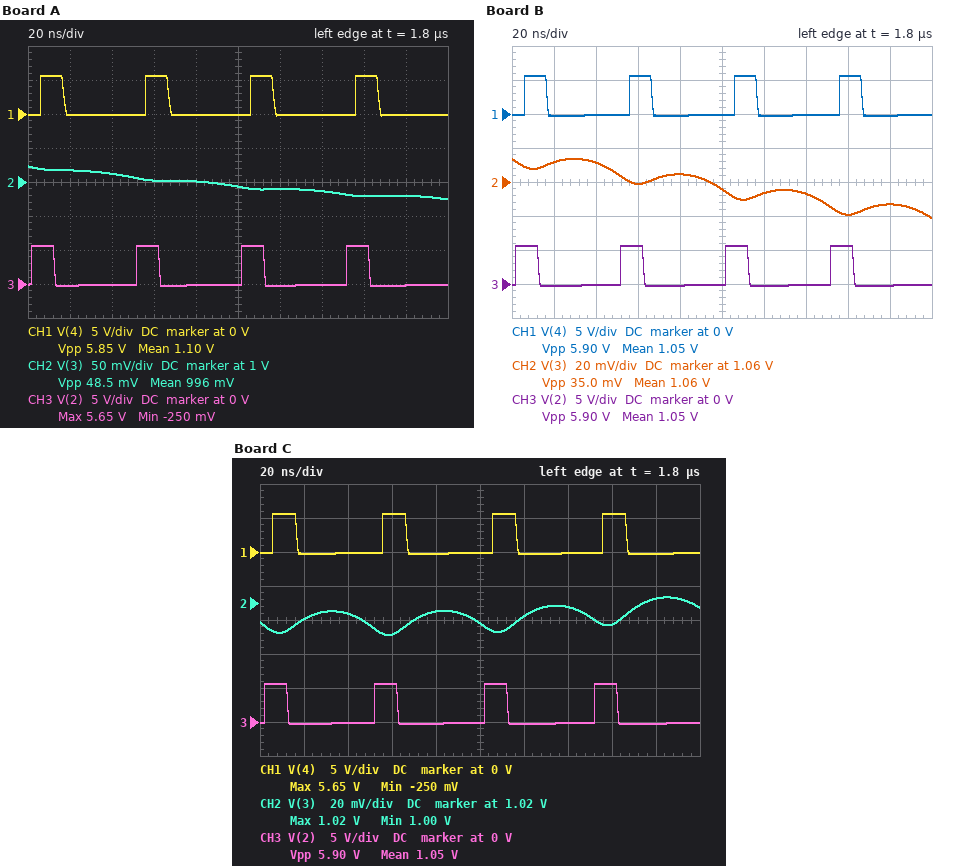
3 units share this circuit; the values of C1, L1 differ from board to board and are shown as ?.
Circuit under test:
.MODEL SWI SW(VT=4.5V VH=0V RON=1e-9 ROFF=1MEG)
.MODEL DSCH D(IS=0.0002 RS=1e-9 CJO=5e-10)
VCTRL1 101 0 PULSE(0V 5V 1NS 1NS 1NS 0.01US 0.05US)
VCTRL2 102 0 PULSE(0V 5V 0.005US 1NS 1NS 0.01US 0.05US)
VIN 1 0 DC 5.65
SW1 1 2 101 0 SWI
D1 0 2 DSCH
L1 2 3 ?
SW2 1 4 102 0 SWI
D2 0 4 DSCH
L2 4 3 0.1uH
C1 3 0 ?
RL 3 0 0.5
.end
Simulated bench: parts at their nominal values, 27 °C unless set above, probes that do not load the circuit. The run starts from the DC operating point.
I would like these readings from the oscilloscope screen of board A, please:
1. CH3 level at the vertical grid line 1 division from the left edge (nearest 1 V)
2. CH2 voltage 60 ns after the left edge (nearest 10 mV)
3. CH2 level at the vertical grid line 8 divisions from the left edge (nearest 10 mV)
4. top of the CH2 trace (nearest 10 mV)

0 V
1.00 V
980 mV
1.02 V
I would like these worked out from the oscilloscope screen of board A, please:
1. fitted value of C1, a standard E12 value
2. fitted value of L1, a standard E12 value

2.7 µF
33 nH
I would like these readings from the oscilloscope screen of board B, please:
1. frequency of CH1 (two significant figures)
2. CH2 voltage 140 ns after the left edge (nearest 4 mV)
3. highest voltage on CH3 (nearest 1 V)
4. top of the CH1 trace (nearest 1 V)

20 MHz
1.052 V
6 V
6 V
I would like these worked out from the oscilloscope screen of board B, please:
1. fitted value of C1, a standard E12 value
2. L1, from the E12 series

680 nF
82 nH
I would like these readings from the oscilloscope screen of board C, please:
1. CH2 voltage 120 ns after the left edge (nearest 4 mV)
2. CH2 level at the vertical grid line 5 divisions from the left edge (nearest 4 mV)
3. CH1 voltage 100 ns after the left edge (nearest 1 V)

1.012 V
1.008 V
0 V
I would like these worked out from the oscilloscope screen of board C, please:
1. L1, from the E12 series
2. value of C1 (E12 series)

47 nH
680 nF
